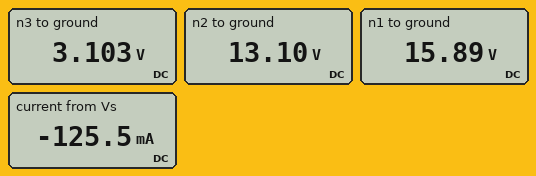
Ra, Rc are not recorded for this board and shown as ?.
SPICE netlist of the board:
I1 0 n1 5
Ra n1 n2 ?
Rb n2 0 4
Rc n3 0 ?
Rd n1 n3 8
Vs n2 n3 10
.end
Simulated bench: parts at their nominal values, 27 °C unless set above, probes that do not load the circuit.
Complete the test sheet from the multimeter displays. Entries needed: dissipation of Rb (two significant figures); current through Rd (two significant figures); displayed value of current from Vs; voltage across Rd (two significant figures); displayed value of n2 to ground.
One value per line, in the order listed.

43 W
1.6 A
-125.5 mA
13 V
13.10 V
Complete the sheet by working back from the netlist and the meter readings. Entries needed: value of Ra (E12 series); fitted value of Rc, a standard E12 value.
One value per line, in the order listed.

0.82 Ω
1.8 Ω
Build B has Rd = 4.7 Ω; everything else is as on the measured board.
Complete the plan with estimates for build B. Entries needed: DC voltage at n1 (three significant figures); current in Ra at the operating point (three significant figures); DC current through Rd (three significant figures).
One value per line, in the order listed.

15.1 V
2.45 A
2.55 A
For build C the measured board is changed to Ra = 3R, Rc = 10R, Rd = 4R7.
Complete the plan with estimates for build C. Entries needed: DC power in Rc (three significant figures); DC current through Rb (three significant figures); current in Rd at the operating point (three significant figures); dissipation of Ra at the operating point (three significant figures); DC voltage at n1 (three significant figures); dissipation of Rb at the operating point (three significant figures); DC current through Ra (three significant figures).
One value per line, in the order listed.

5.10 W
4.29 A
3.25 A
9.22 W
22.4 V
73.5 W
1.75 A
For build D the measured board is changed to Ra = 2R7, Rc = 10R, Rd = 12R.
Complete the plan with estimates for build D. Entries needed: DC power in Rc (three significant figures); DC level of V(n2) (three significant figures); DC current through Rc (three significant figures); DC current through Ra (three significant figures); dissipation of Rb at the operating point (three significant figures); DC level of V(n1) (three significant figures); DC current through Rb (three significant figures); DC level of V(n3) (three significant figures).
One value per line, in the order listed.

5.10 W
17.1 V
714 mA
3.40 A
73.5 W
26.3 V
4.29 A
7.14 V
